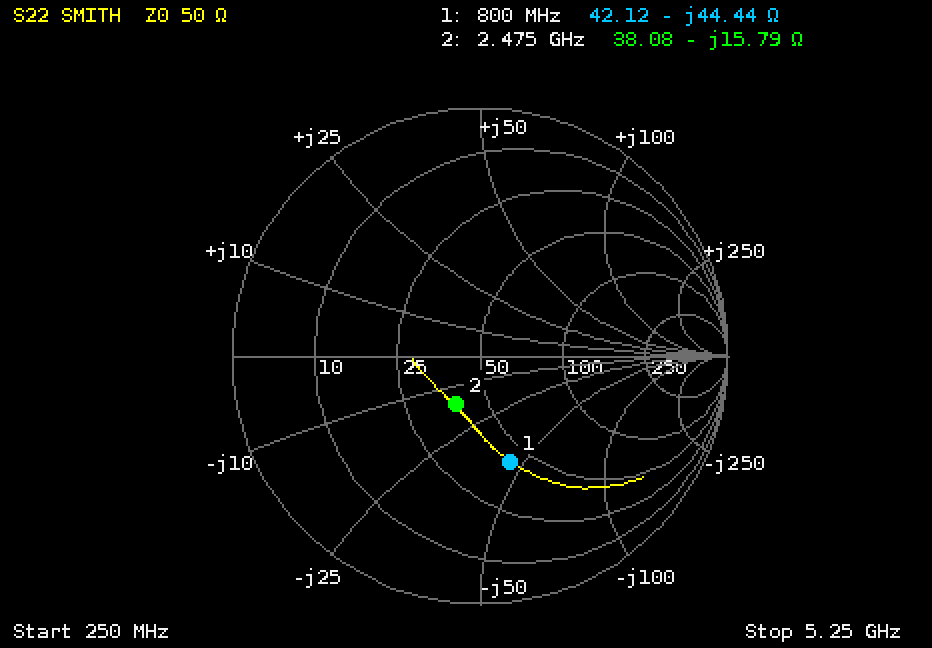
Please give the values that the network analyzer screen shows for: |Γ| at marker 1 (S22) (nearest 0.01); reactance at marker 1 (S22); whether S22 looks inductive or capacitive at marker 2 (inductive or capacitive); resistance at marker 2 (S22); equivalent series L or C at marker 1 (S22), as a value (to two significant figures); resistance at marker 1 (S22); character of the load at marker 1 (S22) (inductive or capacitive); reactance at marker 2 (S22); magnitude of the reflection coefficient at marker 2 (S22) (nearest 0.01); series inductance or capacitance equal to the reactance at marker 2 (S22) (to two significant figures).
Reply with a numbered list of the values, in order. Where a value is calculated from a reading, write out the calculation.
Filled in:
1. 0.44
2. -44.44 Ω
3. capacitive
4. 38.08 Ω
5. C = 1/(2π × 800 MHz × 44.44 Ω) ≈ 4.5 pF
6. 42.12 Ω
7. capacitive
8. -15.79 Ω
9. 0.22
10. C = 1/(2π × 2.475 GHz × 15.79 Ω) ≈ 4.1 pF
